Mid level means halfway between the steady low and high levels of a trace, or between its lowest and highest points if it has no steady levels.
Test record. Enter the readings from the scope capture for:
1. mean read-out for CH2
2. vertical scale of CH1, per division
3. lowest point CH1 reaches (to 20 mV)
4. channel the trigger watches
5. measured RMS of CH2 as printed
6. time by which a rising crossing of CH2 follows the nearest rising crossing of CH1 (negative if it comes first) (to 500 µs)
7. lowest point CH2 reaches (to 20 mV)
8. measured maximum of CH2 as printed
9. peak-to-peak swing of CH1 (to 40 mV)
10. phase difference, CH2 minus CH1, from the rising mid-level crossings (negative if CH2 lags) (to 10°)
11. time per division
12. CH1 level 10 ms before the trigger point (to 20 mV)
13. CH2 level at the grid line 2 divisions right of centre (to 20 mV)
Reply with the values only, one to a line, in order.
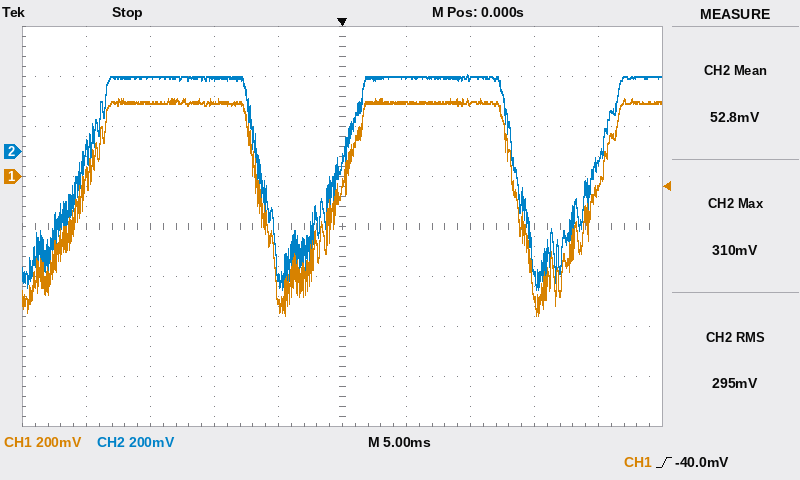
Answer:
52.8 mV
200 mV
-560 mV
CH1
295 mV
0.0 ms
-560 mV
310 mV
880 mV
0°
5 ms
300 mV
300 mV
